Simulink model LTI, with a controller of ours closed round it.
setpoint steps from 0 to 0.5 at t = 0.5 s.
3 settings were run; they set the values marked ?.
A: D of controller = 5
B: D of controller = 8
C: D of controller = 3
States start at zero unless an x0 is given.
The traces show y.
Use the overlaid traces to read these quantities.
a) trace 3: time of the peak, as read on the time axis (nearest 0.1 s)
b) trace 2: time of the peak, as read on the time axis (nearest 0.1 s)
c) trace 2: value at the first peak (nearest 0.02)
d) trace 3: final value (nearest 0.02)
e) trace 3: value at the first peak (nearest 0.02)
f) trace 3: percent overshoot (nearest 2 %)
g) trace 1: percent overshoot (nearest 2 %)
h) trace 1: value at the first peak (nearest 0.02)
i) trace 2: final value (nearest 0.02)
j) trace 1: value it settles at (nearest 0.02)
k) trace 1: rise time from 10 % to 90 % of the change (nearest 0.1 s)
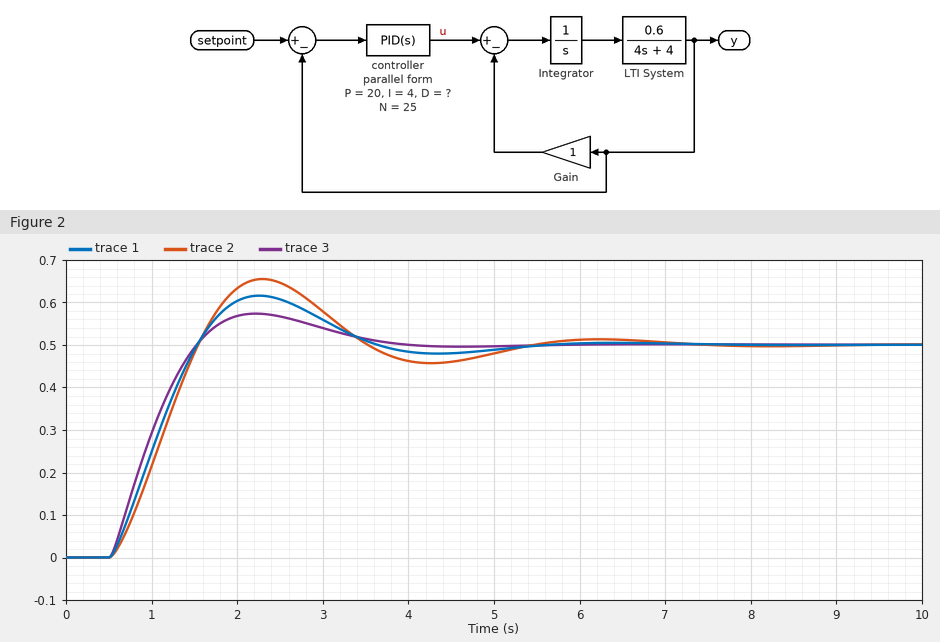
2.2 s
2.3 s
0.66
0.50
0.58
14 %
24 %
0.62
0.50
0.50
0.8 s
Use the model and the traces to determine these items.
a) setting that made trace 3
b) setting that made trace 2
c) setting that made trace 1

B
C
A
